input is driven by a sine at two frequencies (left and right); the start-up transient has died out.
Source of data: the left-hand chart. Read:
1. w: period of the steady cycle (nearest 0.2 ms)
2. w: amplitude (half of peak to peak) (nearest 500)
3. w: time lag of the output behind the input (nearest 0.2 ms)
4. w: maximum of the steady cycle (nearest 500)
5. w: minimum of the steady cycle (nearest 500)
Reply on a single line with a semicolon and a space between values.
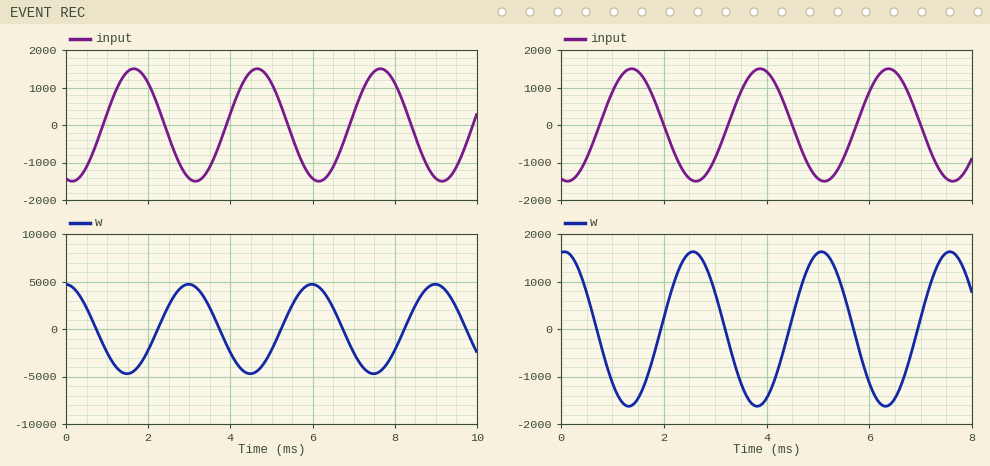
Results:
3.0 ms; 4500; 1.4 ms; 4500; -4500
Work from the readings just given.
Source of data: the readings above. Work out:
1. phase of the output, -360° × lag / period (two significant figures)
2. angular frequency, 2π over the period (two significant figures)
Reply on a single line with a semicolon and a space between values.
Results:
-170°; 2.1 rad/ms
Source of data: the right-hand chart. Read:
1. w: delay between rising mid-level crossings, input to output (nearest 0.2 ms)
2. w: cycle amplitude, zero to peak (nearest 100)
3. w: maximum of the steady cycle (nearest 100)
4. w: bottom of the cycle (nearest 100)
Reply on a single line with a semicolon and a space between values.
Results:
1.2 ms; 1600; 1600; -1600
